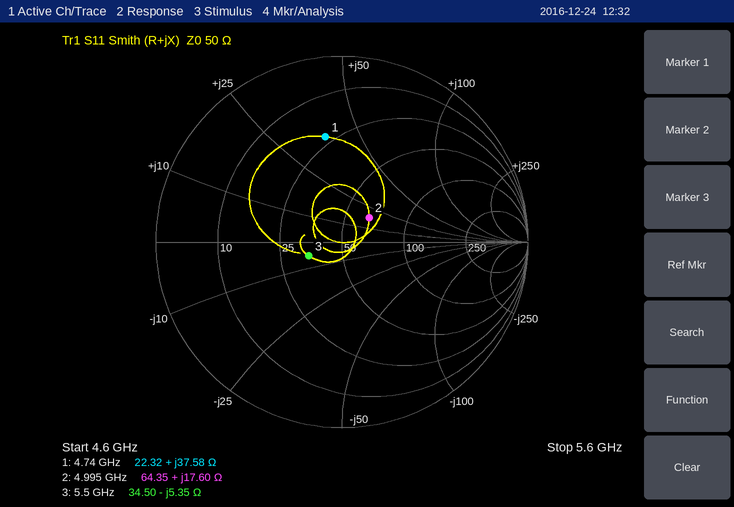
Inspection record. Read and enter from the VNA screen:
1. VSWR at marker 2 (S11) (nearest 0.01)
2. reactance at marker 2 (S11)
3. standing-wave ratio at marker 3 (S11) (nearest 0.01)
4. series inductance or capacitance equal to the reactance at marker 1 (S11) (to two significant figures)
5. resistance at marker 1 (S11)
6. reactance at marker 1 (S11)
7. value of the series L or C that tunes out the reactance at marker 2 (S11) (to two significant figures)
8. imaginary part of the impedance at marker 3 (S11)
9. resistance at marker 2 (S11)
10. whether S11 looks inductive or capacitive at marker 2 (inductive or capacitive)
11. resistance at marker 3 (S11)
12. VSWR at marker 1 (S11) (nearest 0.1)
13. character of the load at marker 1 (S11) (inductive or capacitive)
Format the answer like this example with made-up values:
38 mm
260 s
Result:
1.49
+17.60 Ω
1.48
1.3 nH
22.32 Ω
+37.58 Ω
1.8 pF
-5.35 Ω
64.35 Ω
inductive
34.50 Ω
3.7
inductive
